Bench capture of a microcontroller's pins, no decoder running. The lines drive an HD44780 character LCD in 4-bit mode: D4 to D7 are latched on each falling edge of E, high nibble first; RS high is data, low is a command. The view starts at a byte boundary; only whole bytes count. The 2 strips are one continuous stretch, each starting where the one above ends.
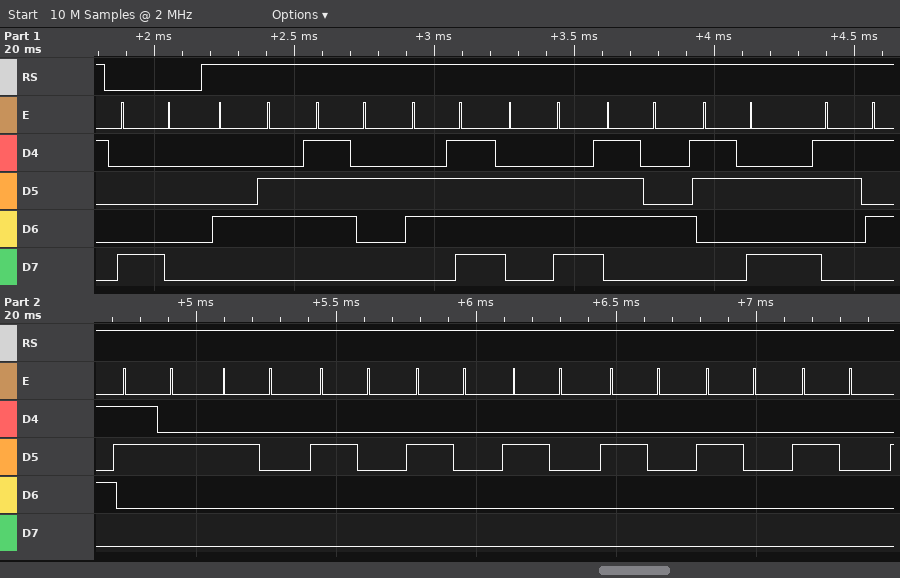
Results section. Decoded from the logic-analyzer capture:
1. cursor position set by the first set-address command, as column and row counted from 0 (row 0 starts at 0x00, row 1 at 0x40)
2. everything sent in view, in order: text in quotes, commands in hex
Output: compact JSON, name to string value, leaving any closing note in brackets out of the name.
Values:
{"cursor position set by the first set-address command, as column and row counted from 0": "column 0, row 0", "everything sent in view, in order: text in quotes, commands in hex": "0x80 \"Front:52       \""}
